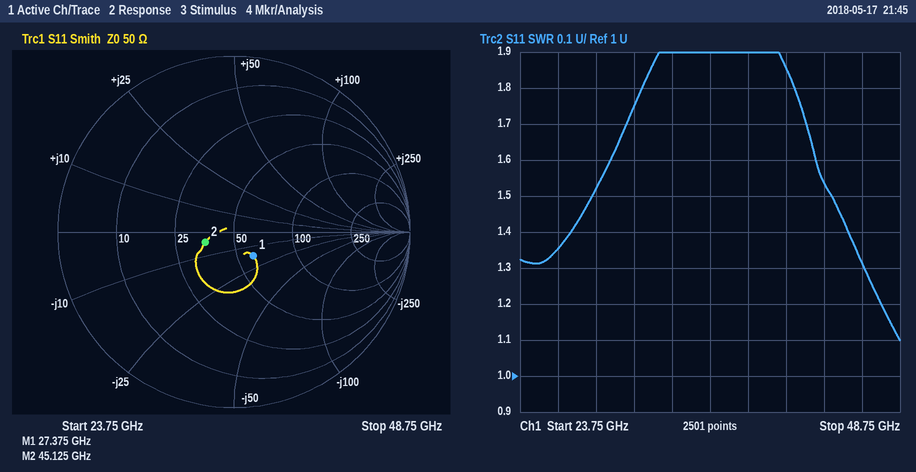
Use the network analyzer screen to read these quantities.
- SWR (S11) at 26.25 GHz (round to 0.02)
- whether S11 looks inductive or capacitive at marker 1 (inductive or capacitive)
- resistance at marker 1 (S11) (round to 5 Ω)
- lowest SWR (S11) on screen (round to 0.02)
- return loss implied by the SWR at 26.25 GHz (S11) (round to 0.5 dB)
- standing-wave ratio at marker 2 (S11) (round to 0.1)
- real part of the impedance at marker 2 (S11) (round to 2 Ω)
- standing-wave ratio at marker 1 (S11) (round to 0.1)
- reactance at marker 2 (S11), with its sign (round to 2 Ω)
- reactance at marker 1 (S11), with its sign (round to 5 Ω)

1.36
capacitive
60 Ω
1.10
16.5 dB
1.4
36 Ω
1.4
-4 Ω
-15 Ω
